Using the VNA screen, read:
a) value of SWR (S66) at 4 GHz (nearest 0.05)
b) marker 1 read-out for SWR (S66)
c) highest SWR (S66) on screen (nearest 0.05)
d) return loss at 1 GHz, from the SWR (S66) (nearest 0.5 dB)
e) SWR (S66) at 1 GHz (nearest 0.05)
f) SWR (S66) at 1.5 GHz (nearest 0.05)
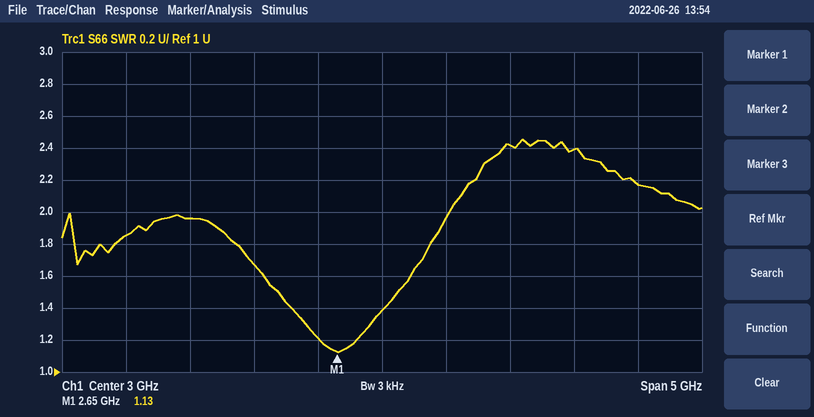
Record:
2.40
1.13
2.45
10.5 dB
1.85
1.95
